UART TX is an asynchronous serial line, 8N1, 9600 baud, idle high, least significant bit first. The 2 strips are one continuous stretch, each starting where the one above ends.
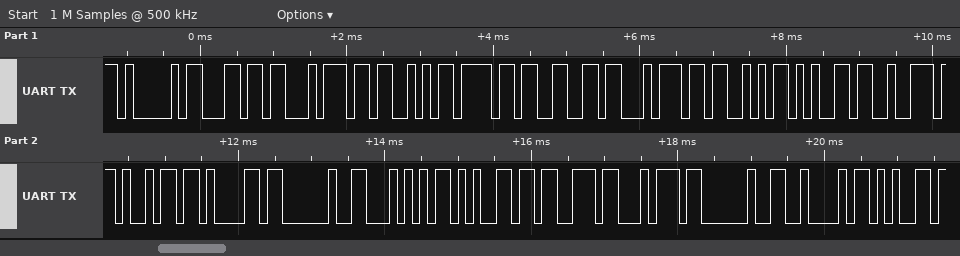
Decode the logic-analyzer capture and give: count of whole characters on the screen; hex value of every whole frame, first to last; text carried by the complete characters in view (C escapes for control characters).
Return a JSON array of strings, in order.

["20", "0x41 0x6C 0x74 0x53 0x6F 0x66 0x74 0x53 0x65 0x72 0x69 0x61 0x20 0x54 0x65 0x73 0x74 0x20 0x42 0x65", "\"AltSoftSeria Test Be\""]
